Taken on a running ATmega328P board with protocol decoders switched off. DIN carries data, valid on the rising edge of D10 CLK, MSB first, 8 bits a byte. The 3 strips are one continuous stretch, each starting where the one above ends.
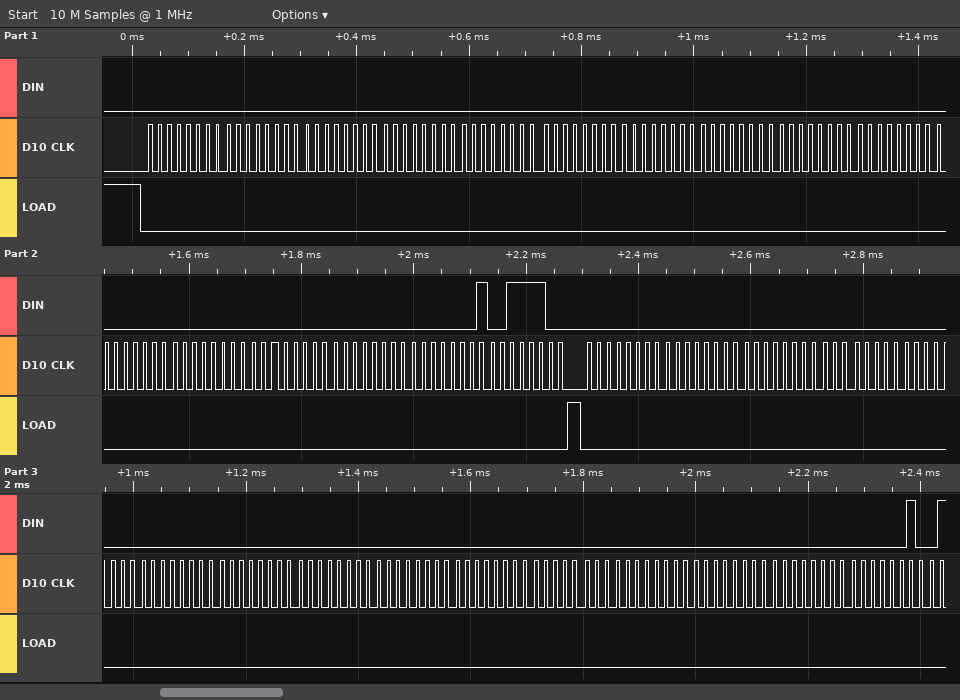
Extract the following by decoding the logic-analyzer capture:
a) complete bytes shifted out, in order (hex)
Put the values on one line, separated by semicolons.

0x00 0x00 0x00 0x00 0x00 0x00 0x00 0x00 0x00 0x00 0x00 0x00 0x00 0x00 0x01 0x3C 0x00 0x00 0x00 0x00 0x00 0x00 0x00 0x00 0x00 0x00 0x00 0x00 0x00 0x00 0x02
